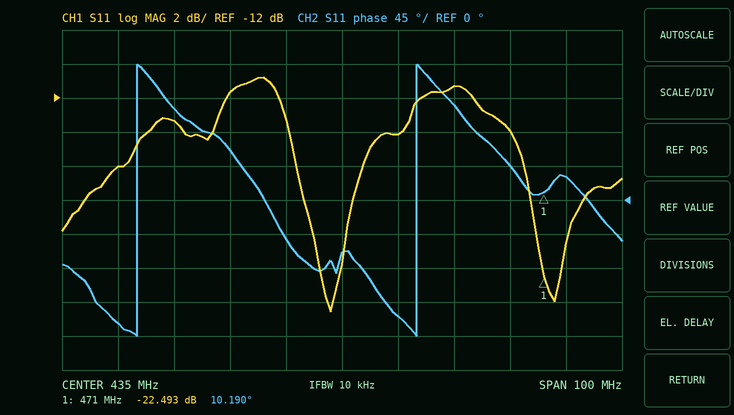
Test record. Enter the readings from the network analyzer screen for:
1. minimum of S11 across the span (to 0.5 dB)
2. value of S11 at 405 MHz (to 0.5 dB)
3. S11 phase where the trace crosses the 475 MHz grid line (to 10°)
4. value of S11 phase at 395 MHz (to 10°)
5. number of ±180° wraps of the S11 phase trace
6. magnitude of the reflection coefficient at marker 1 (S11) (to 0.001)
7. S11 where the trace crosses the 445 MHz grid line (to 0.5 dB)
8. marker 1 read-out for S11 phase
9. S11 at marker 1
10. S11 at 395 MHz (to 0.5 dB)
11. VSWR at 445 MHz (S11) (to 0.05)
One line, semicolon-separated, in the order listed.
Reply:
-24.5 dB; -13.5 dB; 30°; -160°; 2; 0.075; -14.0 dB; 10.190°; -22.493 dB; -16.0 dB; 1.50
